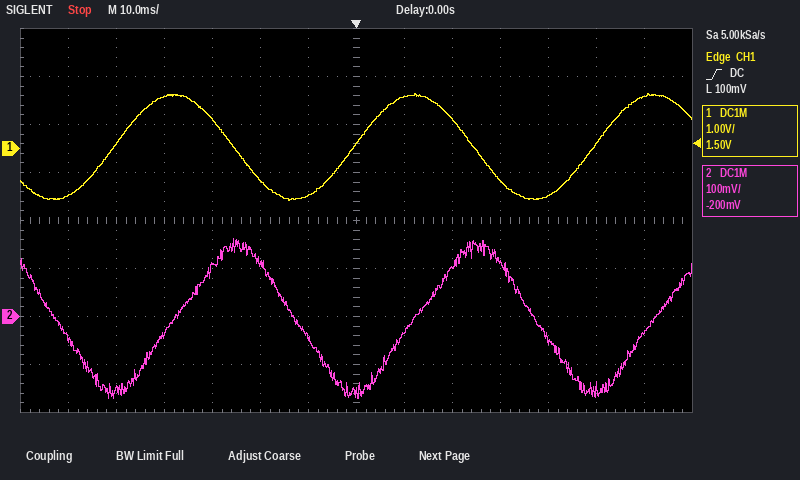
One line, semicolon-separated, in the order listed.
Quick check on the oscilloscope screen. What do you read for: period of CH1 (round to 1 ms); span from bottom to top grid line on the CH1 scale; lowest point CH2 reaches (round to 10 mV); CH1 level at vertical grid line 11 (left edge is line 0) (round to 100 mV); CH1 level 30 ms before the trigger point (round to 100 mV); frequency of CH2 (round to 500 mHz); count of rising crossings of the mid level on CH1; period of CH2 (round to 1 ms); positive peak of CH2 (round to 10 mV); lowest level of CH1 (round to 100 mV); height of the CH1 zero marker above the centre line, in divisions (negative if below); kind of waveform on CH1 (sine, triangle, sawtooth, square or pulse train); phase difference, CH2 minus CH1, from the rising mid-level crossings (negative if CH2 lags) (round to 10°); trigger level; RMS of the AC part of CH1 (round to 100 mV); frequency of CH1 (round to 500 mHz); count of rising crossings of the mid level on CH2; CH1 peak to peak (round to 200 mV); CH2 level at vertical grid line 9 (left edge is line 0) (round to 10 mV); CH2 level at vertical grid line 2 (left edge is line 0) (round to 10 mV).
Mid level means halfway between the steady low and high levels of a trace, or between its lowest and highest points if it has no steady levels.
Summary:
50 ms; 8 V; -170 mV; -1.0 V; 600 mV; 20.0 Hz; 3; 50 ms; 160 mV; -1.1 V; +1.5 div; sine; -90°; 100 mV; 800 mV; 20.0 Hz; 3; 2.2 V; 100 mV; -150 mV
